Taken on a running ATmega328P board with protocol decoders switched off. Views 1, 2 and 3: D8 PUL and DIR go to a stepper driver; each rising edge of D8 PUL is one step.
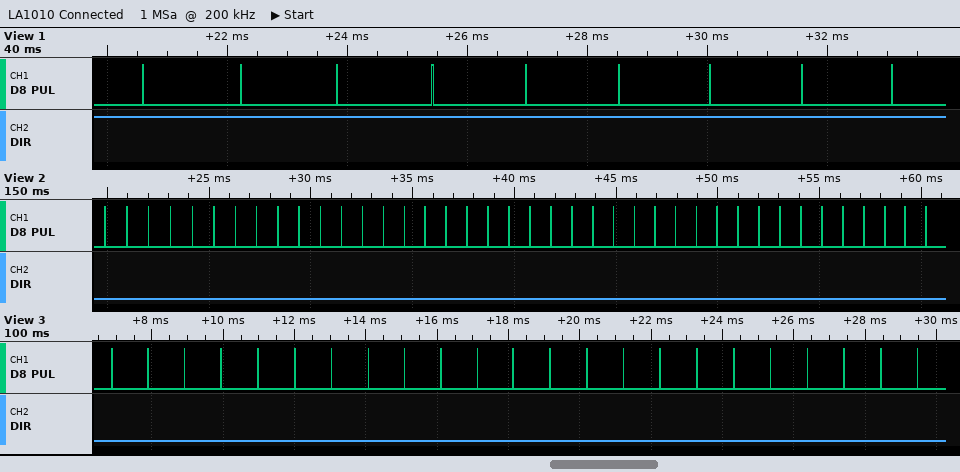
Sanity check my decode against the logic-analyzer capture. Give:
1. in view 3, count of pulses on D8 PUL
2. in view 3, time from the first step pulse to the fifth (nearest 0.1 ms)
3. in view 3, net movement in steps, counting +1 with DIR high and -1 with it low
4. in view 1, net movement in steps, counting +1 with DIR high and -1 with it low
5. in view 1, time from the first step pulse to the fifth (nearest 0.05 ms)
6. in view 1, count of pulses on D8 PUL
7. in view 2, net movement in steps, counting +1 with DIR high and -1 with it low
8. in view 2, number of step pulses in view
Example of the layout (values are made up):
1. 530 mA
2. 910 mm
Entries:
1. 23
2. 4.1 ms
3. -23
4. +9
5. 6.35 ms
6. 9
7. -40
8. 40
